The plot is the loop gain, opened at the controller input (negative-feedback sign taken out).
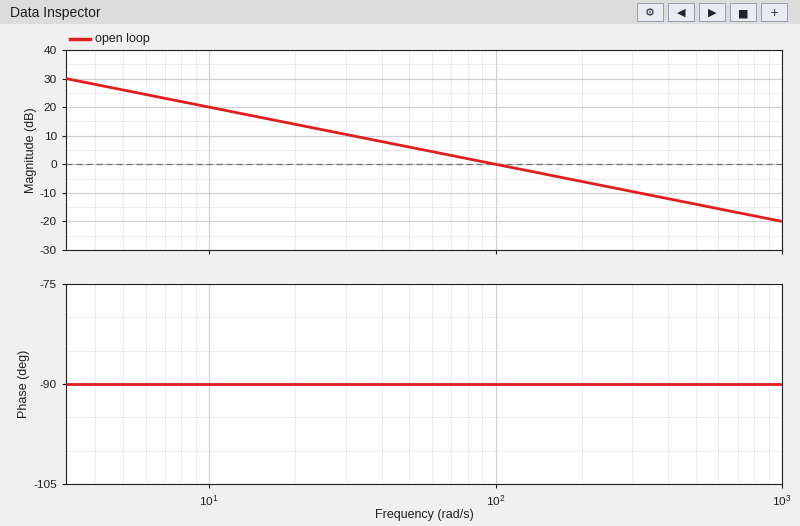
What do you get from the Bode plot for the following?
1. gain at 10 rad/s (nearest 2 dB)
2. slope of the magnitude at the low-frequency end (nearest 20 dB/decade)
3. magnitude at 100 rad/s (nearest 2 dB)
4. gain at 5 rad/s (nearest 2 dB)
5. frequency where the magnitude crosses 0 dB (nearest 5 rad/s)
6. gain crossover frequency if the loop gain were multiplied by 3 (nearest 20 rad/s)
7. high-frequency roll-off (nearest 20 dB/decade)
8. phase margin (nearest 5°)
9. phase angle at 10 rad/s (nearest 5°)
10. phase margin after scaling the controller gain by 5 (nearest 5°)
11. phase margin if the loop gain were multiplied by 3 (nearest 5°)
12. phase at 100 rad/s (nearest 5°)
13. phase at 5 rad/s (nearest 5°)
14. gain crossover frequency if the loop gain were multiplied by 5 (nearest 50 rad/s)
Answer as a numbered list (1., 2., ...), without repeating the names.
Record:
1. 20 dB
2. -20 dB/decade
3. 0 dB
4. 26 dB
5. 100 rad/s
6. 300 rad/s
7. -20 dB/decade
8. 90°
9. -90°
10. 90°
11. 90°
12. -90°
13. -90°
14. 500 rad/s
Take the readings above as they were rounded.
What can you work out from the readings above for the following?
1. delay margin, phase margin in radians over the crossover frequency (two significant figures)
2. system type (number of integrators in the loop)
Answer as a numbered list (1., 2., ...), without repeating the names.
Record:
1. 0.016 s
2. 1
